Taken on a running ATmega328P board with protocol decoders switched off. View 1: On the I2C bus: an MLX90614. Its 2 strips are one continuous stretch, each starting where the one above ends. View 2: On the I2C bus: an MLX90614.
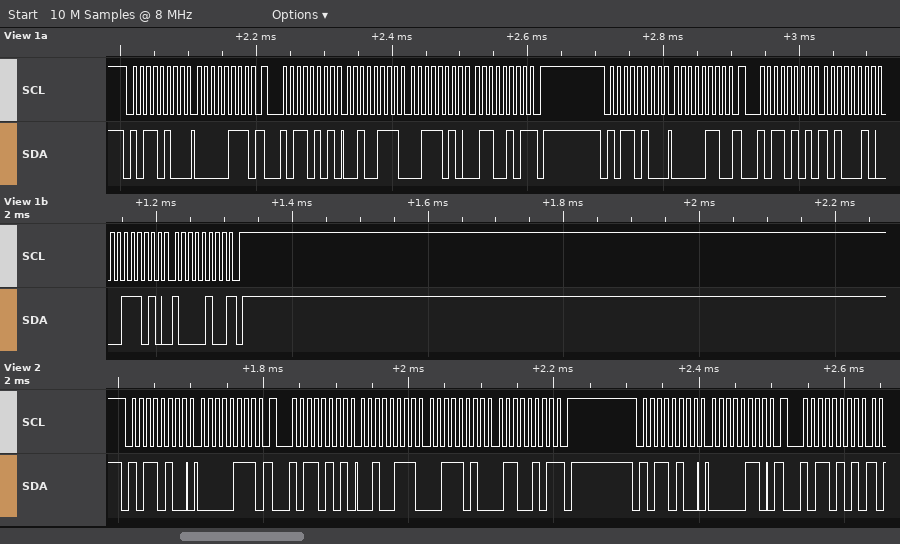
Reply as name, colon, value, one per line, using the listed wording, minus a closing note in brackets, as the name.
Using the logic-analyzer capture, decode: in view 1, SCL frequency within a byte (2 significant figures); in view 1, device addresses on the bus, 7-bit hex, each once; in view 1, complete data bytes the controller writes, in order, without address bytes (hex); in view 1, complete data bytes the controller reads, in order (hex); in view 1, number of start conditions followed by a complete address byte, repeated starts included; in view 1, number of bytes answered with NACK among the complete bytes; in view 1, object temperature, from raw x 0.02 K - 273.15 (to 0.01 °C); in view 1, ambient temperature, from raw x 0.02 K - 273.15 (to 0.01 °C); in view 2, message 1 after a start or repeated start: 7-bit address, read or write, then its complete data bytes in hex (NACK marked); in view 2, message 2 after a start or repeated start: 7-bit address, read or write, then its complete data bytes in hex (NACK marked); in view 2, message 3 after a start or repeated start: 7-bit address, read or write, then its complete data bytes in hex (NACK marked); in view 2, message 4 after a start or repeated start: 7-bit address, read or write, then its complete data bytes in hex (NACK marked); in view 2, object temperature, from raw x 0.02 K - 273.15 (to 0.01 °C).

in view 1, SCL frequency within a byte: 100 kHz
in view 1, device addresses on the bus, 7-bit hex, each once: 0x5A
in view 1, complete data bytes the controller writes, in order, without address bytes: 07 06
in view 1, complete data bytes the controller reads, in order: 27 3A 65 A2 3A 84
in view 1, number of start conditions followed by a complete address byte, repeated starts included: 4
in view 1, number of bytes answered with NACK among the complete bytes: 2
in view 1, object temperature, from raw x 0.02 K - 273.15: 24.59 °C
in view 1, ambient temperature, from raw x 0.02 K - 273.15: 27.05 °C
in view 2, message 1 after a start or repeated start: 7-bit address, read or write, then its complete data bytes in hex: 0x5A write: 07
in view 2, message 2 after a start or repeated start: 7-bit address, read or write, then its complete data bytes in hex: 0x5A read: 27 3A 65 NACK
in view 2, message 3 after a start or repeated start: 7-bit address, read or write, then its complete data bytes in hex: 0x5A write: 06
in view 2, message 4 after a start or repeated start: 7-bit address, read or write, then its complete data bytes in hex: 0x5A read
in view 2, object temperature, from raw x 0.02 K - 273.15: 24.59 °C
